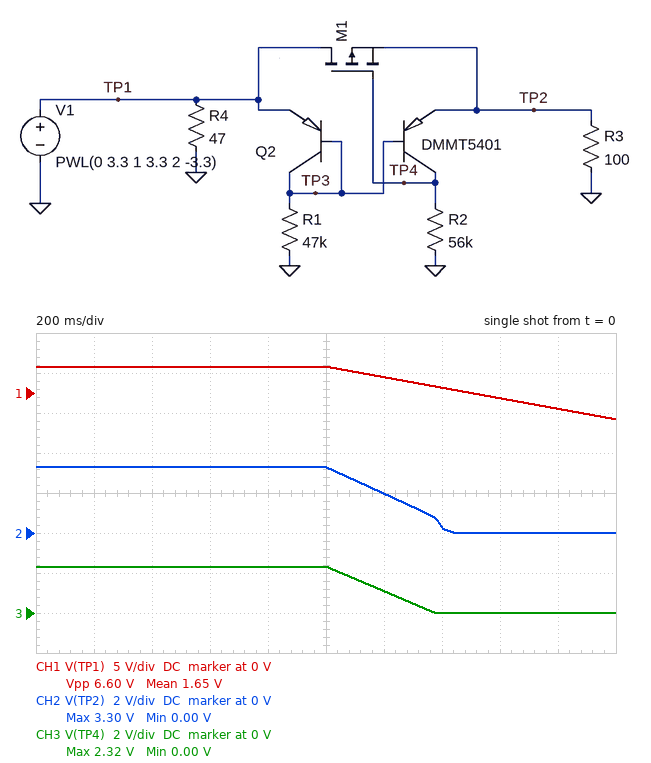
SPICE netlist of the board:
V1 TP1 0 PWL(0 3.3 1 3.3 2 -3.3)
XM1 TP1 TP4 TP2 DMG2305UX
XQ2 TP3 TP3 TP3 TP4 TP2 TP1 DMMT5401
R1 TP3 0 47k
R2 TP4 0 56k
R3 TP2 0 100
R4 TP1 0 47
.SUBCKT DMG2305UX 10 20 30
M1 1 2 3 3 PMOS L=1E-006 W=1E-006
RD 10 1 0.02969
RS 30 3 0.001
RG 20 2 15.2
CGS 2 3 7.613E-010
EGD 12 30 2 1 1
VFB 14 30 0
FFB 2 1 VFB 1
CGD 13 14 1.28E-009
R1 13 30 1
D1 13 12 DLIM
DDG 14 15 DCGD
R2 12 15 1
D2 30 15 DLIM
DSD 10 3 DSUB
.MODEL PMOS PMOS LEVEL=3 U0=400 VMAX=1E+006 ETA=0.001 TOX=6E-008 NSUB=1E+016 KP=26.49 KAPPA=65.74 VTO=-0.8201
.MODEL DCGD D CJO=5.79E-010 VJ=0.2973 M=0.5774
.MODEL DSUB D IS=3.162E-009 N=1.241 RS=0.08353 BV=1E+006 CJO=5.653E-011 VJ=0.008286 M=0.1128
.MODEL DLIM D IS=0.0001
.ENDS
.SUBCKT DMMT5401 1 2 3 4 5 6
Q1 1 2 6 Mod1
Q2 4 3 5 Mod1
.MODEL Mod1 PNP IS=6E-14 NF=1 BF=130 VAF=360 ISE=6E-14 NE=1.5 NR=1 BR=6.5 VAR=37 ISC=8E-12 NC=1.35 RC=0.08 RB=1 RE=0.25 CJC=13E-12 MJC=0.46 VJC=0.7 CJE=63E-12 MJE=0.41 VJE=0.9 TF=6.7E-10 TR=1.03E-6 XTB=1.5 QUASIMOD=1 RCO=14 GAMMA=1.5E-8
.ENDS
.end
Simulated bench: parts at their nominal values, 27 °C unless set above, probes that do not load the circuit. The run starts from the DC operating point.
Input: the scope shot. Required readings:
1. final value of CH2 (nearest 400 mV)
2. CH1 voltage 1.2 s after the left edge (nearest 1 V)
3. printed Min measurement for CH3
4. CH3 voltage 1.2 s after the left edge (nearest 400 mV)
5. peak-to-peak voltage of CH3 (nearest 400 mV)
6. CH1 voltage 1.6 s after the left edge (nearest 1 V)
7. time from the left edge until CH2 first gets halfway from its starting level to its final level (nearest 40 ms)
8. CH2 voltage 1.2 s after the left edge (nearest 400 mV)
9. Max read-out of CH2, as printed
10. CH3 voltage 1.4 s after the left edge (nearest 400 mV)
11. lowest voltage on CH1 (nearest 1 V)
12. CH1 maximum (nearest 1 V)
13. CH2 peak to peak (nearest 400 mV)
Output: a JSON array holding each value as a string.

["0 V", "2 V", "0.00 V", "1.2 V", "2.4 V", "-1 V", "1.24 s", "2.0 V", "3.30 V", "0 V", "-3 V", "3 V", "3.2 V"]
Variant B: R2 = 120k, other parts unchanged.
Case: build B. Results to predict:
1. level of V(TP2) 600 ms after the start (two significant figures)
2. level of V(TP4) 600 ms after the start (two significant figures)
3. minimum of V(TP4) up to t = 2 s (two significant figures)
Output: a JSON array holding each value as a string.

["3.3 V", "2.4 V", "-3.0 mV"]
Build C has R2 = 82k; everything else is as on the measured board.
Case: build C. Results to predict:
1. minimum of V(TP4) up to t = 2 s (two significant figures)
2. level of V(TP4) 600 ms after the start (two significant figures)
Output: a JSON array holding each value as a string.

["-2.0 mV", "2.4 V"]
